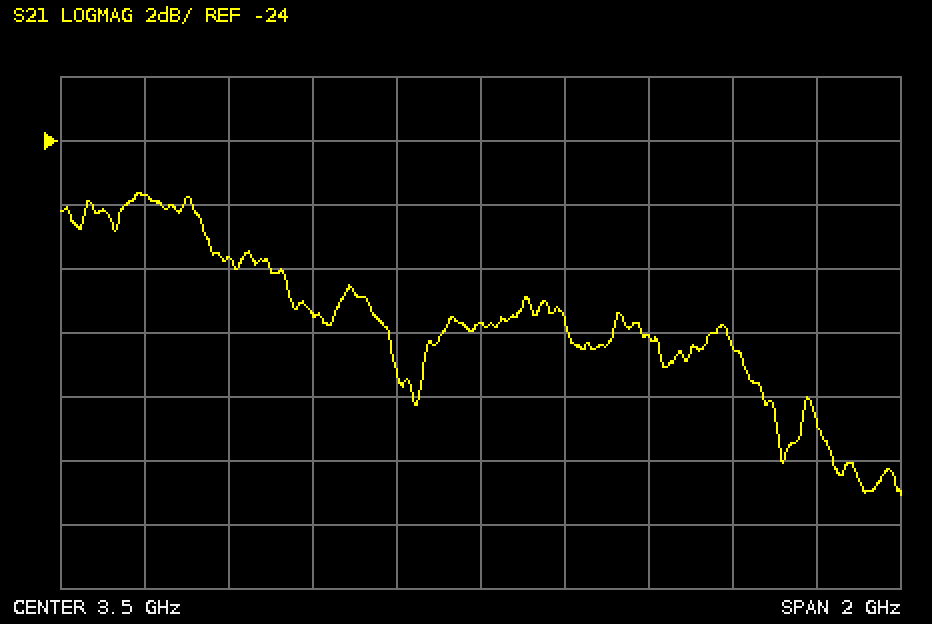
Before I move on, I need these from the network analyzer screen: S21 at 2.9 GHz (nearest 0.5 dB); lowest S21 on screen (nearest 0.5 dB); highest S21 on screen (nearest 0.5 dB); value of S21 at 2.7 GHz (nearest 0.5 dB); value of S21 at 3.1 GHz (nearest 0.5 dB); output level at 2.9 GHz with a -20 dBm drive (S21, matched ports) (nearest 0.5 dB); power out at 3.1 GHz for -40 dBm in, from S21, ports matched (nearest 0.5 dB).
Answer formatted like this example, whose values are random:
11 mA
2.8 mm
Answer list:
-27.5 dB
-35.0 dB
-25.5 dB
-25.5 dB
-29.5 dB
-47.5 dBm
-69.5 dBm
